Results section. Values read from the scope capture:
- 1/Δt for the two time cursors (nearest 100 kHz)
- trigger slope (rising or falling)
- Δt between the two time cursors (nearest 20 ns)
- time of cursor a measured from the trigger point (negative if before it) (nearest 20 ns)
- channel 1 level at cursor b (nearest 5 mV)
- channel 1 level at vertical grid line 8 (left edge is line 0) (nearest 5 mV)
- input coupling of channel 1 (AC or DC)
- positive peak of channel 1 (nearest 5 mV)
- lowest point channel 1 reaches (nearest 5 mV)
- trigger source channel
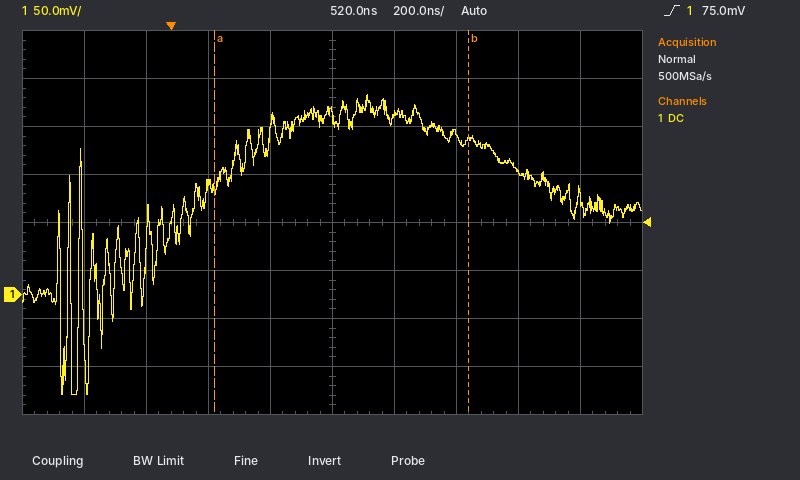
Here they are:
1.2 MHz
rising
820 ns
+140 ns
160 mV
130 mV
DC
210 mV
-105 mV
channel 1
